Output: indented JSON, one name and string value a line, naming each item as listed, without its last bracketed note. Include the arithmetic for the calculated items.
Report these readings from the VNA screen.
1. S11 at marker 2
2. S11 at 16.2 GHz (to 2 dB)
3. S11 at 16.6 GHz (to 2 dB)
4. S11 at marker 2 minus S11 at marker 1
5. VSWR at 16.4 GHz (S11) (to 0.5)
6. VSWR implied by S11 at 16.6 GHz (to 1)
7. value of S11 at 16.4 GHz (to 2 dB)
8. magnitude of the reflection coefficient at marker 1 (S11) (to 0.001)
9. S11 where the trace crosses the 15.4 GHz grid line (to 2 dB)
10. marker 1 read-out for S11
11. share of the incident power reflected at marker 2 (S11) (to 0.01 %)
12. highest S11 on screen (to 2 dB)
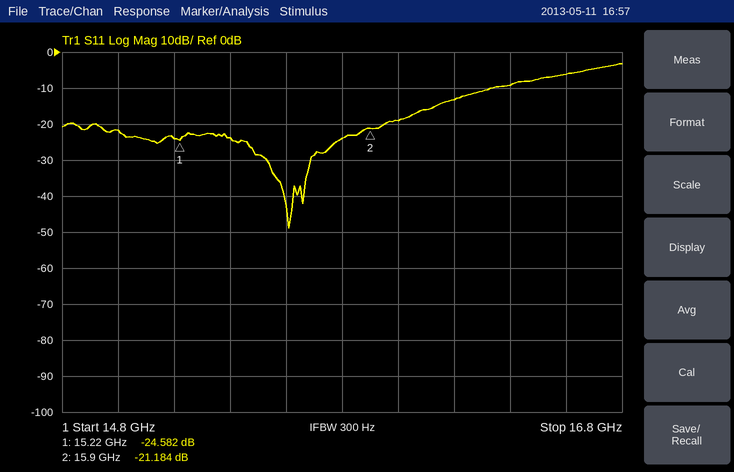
{
  "S11 at marker 2": "-21.184 dB",
  "S11 at 16.2 GHz": "-14 dB",
  "S11 at 16.6 GHz": "-6 dB",
  "S11 at marker 2 minus S11 at marker 1": "-21.184 − (-24.582) = 3.398 dB",
  "VSWR at 16.4 GHz (S11)": "|Γ| = 10^(-10/20) = 0.3162; VSWR = (1 + 0.3162)/(1 − 0.3162) ≈ 1.92, so 2.0 to the nearest 0.5",
  "VSWR implied by S11 at 16.6 GHz": "|Γ| = 10^(-6/20) = 0.5012; VSWR = (1 + 0.5012)/(1 − 0.5012) ≈ 3",
  "value of S11 at 16.4 GHz": "-10 dB",
  "magnitude of the reflection coefficient at marker 1 (S11)": "10^(-24.582/20) ≈ 0.059",
  "S11 where the trace crosses the 15.4 GHz grid line": "-24 dB",
  "marker 1 read-out for S11": "-24.582 dB",
  "share of the incident power reflected at marker 2 (S11)": "10^(-21.184/10) ≈ 0.76 %",
  "highest S11 on screen": "-4 dB"
}
